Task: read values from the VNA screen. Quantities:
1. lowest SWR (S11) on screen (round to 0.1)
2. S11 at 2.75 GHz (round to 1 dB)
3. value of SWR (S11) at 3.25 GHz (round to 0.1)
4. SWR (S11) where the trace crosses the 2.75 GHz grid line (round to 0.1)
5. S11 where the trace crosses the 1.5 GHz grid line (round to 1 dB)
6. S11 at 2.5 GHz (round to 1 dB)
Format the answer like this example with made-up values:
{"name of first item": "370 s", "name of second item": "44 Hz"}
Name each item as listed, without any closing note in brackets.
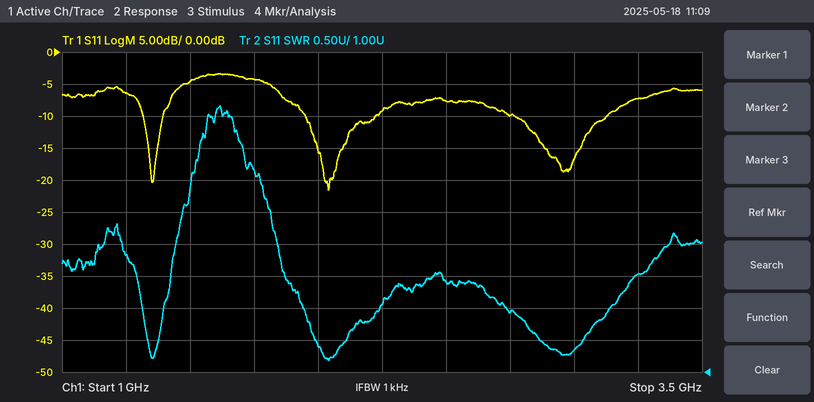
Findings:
{"lowest SWR (S11) on screen": "1.2", "S11 at 2.75 GHz": "-10 dB", "value of SWR (S11) at 3.25 GHz": "2.5", "SWR (S11) where the trace crosses the 2.75 GHz grid line": "1.9", "S11 where the trace crosses the 1.5 GHz grid line": "-5 dB", "S11 at 2.5 GHz": "-8 dB"}
